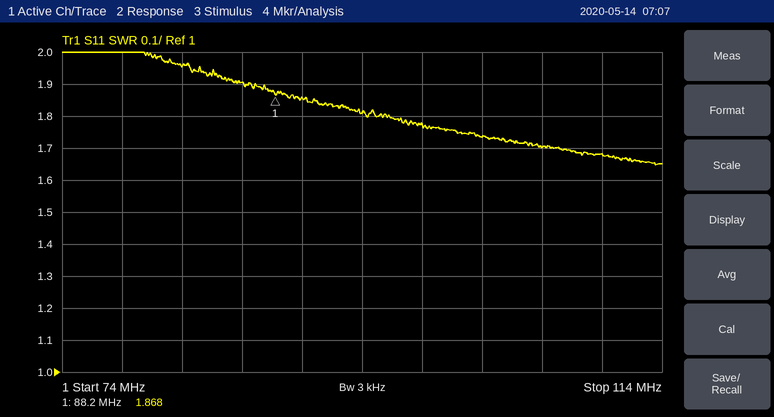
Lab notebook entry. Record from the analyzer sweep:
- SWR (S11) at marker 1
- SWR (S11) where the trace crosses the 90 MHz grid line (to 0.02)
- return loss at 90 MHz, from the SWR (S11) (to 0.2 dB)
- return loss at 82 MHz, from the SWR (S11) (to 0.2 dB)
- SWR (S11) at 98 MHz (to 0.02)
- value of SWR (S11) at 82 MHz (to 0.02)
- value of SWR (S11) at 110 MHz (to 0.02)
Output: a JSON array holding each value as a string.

["1.868", "1.86", "10.4 dB", "9.8 dB", "1.78", "1.96", "1.68"]
